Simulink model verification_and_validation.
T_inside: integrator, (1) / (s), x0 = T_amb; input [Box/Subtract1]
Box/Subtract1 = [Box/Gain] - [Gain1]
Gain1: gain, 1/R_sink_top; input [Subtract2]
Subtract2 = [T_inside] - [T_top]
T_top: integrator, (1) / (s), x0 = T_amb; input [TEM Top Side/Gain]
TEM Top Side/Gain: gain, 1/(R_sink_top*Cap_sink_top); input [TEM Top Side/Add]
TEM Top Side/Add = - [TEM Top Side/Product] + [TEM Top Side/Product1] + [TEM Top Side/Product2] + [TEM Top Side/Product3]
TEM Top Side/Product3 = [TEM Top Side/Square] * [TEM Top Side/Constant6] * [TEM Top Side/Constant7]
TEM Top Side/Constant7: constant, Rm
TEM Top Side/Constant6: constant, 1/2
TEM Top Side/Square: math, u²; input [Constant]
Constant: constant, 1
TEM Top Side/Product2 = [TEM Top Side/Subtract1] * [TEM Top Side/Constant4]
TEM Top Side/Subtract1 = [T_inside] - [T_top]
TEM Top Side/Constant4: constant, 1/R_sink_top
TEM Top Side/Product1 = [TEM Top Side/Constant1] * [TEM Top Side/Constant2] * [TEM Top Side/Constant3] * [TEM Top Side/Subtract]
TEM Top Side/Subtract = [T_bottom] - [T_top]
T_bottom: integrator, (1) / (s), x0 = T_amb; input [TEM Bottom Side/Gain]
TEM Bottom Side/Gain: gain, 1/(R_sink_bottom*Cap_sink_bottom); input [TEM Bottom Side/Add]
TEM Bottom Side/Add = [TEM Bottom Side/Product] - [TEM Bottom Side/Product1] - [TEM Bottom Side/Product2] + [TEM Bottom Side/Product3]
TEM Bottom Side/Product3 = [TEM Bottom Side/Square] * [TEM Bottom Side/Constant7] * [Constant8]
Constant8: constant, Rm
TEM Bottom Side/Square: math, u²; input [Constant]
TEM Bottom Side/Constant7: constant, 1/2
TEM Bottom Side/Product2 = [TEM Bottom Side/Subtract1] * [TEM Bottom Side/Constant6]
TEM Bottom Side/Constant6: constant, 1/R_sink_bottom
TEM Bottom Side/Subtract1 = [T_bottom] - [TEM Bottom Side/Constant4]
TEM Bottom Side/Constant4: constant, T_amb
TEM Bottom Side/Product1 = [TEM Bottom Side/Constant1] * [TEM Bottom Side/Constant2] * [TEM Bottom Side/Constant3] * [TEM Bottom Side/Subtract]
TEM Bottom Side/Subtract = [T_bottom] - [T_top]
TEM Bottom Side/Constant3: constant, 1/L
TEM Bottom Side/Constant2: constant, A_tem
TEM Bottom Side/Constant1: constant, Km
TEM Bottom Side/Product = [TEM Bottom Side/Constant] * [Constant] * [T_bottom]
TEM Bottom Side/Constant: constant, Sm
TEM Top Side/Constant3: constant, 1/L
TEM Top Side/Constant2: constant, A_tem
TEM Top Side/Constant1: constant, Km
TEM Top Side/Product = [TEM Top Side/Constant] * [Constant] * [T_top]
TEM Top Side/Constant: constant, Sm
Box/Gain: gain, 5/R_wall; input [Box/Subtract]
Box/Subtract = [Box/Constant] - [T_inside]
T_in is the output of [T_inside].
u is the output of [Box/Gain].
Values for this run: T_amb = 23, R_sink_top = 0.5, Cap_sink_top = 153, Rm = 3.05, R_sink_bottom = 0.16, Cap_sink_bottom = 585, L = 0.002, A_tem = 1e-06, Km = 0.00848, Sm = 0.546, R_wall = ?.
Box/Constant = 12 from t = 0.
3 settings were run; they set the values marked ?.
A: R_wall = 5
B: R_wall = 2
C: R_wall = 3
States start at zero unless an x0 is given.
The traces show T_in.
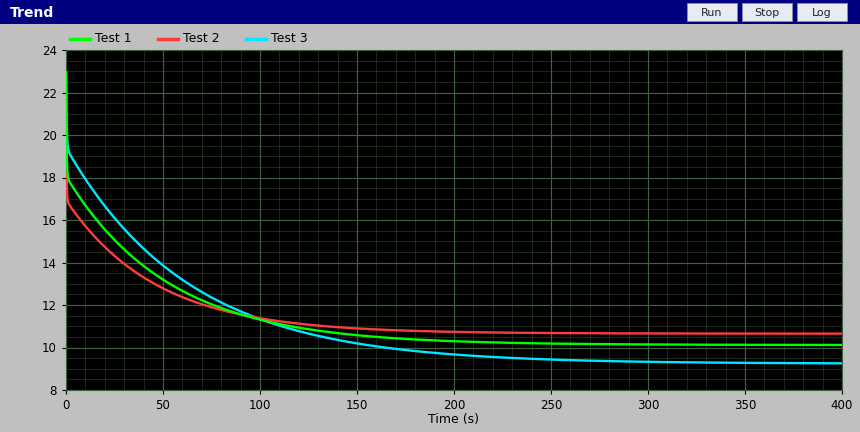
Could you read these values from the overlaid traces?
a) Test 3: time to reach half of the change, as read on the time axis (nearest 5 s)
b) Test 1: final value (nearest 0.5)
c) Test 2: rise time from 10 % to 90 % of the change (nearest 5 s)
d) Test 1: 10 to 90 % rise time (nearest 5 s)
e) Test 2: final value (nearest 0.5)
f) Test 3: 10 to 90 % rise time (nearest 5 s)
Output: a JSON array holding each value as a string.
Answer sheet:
["25 s", "10.0", "75 s", "95 s", "10.5", "125 s"]
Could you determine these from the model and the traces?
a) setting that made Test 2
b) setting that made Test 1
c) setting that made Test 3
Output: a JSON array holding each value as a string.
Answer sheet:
["B", "C", "A"]
